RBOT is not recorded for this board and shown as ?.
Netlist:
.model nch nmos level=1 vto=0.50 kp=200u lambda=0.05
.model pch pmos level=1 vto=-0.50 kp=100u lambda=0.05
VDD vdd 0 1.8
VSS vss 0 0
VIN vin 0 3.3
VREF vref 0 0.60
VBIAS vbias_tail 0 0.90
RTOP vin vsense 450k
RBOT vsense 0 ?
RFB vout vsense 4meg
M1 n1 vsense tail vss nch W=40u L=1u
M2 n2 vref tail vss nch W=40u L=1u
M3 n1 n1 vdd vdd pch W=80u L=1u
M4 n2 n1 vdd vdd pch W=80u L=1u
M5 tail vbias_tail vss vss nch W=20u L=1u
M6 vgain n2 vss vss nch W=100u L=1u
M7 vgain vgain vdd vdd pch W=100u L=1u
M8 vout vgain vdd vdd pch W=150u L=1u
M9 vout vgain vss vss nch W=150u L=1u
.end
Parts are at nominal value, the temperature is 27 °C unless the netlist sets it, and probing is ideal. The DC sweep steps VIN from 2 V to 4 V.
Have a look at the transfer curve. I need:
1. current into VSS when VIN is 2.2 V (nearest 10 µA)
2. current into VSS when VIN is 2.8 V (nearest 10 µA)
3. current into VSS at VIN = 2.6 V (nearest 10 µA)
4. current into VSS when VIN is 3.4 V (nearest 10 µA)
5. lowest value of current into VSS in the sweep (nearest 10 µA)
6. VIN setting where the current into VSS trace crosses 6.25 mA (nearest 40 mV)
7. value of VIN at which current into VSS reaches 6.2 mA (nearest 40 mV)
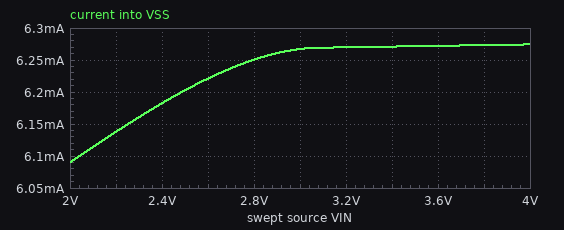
6.14 mA
6.25 mA
6.22 mA
6.27 mA
6.09 mA
2.80 V
2.48 V
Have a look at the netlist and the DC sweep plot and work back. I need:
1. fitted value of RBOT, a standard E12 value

270 kΩ
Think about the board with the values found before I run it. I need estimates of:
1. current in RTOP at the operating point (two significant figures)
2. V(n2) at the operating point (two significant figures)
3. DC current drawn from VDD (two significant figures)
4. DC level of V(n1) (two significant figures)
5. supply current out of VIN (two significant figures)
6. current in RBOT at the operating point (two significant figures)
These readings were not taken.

4.5 µA
1.8 V
6.3 mA
1.0 V
4.5 µA
4.7 µA
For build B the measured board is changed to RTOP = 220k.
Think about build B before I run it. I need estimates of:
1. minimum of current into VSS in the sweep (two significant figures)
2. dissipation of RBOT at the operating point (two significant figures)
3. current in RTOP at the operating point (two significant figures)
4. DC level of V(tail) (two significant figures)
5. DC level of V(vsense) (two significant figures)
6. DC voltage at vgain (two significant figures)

6.3 mA
12 µW
6.7 µA
900 mV
1.8 V
250 mV
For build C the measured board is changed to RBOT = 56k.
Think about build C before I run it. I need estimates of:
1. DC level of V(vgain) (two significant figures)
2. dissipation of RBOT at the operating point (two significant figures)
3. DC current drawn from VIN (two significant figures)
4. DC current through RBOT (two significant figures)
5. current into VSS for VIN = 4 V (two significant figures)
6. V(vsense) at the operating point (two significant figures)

1.3 V
2.3 µW
6.5 µA
6.4 µA
110 nA
360 mV
